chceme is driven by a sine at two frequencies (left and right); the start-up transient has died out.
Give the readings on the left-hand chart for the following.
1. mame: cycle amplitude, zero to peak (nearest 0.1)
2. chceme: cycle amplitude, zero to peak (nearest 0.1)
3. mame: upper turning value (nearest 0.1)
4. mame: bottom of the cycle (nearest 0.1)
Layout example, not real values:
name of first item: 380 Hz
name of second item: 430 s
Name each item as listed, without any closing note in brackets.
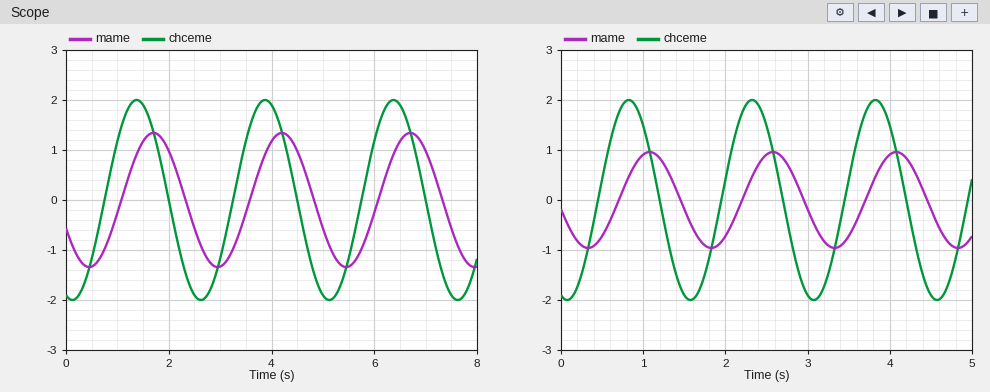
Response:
mame: cycle amplitude, zero to peak: 1.3
chceme: cycle amplitude, zero to peak: 2.0
mame: upper turning value: 1.3
mame: bottom of the cycle: -1.3
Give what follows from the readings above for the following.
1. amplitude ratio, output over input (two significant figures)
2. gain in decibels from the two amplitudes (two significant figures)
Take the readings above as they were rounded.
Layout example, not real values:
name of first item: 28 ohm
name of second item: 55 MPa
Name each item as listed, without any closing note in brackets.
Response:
amplitude ratio, output over input: 0.65
gain in decibels from the two amplitudes: -3.7 dB
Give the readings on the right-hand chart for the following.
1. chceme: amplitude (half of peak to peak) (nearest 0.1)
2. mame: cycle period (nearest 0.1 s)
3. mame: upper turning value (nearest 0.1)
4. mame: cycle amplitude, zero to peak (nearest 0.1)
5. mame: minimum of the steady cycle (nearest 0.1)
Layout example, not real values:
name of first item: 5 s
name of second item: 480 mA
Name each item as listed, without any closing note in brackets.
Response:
chceme: amplitude (half of peak to peak): 2.0
mame: cycle period: 1.5 s
mame: upper turning value: 1.0
mame: cycle amplitude, zero to peak: 1.0
mame: minimum of the steady cycle: -1.0
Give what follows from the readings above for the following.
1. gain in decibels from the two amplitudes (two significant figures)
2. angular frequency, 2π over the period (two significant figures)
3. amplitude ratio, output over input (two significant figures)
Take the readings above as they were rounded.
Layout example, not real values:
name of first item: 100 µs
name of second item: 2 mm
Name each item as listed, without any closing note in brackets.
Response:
gain in decibels from the two amplitudes: -6.0 dB
angular frequency, 2π over the period: 4.2 rad/s
amplitude ratio, output over input: 0.50
